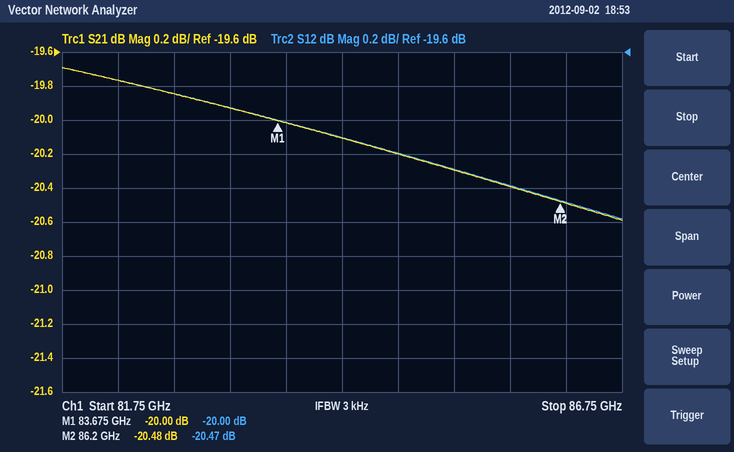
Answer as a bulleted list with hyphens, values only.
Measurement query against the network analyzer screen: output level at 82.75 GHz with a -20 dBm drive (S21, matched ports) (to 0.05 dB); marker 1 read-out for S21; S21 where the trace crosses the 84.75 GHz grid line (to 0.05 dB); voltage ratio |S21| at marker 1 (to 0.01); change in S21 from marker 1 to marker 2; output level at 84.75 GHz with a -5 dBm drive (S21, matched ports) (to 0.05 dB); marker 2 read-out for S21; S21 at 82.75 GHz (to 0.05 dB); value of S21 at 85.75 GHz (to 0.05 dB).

- -39.85 dBm
- -20.00 dB
- -20.20 dB
- 0.10
- -0.48 dB
- -25.20 dBm
- -20.48 dB
- -19.85 dB
- -20.40 dB
